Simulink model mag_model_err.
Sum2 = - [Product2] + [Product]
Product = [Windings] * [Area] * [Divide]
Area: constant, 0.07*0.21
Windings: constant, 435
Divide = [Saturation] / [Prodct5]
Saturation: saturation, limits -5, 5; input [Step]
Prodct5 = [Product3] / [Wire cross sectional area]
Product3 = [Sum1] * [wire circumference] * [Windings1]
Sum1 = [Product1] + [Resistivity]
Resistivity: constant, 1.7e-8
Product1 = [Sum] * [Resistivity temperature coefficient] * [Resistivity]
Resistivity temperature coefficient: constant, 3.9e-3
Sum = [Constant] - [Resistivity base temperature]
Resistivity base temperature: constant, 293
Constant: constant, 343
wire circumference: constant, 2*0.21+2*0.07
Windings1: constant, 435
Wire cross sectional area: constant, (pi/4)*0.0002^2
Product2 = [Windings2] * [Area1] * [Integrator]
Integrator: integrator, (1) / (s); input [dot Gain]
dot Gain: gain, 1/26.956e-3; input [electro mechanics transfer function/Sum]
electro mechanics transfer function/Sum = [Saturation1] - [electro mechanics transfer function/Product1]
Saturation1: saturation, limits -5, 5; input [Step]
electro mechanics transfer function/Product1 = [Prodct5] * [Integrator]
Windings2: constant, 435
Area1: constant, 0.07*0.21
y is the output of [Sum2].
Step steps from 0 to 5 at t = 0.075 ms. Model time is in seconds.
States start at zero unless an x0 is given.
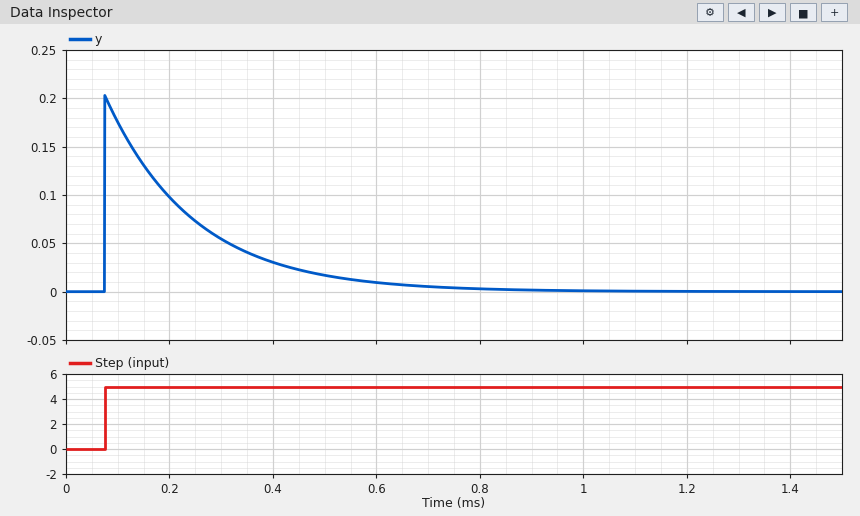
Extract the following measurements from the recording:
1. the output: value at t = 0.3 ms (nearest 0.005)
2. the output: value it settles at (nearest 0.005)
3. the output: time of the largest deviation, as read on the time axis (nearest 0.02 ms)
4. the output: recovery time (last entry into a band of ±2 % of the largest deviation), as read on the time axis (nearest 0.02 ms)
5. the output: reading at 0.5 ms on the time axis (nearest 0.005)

0.055
0.000
0.08 ms
0.74 ms
0.015
